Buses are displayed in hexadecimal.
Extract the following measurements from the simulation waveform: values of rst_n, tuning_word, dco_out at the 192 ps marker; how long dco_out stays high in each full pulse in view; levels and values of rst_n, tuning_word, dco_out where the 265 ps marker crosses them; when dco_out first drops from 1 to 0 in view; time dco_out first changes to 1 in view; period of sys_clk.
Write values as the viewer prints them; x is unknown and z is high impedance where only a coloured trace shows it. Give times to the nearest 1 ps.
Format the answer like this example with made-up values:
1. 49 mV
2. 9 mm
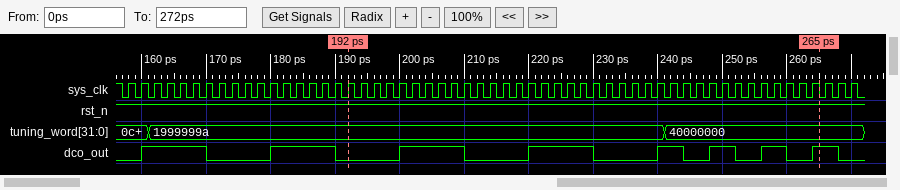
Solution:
1. rst_n=1, tuning_word=1999999a, dco_out=0
2. 10 ps, 10 ps, 10 ps, 10 ps, 4 ps, 4 ps, 4 ps, 4 ps
3. rst_n=1, tuning_word=40000000, dco_out=1
4. 170 ps
5. 160 ps
6. 2 ps
